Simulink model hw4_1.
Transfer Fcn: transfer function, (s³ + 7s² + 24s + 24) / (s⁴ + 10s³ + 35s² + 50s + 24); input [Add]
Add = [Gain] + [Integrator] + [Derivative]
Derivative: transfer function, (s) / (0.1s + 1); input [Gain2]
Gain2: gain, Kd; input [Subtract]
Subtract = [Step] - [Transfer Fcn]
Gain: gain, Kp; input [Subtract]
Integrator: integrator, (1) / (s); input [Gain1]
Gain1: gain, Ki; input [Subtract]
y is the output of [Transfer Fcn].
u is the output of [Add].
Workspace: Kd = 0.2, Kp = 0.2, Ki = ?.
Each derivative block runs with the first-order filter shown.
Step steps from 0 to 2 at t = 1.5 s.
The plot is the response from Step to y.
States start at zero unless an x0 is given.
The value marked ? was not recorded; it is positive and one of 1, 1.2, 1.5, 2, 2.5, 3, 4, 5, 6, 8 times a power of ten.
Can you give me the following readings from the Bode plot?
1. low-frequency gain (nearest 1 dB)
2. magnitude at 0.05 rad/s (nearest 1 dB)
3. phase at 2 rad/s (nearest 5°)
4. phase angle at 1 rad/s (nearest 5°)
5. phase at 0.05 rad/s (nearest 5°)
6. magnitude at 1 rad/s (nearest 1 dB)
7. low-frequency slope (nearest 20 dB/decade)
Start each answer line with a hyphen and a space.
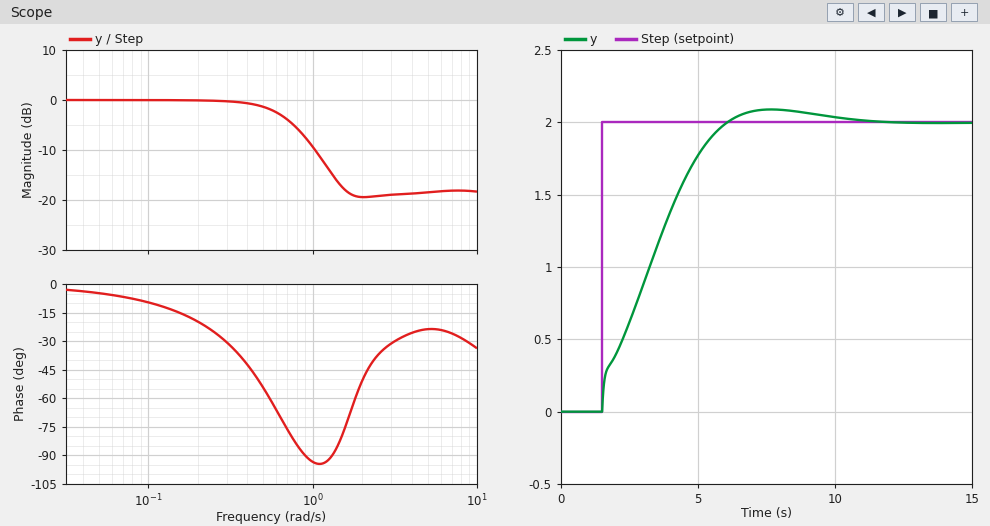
- 0 dB
- 0 dB
- -50°
- -95°
- -5°
- -9 dB
- 0 dB/decade
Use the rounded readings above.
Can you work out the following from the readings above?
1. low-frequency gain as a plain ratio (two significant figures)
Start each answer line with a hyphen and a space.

- 1.0
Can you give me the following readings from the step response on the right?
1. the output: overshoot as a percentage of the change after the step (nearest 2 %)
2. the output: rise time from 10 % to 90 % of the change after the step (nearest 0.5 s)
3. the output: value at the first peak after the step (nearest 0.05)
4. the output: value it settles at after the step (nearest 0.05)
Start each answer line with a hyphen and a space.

- 4 %
- 3.5 s
- 2.10
- 2.00
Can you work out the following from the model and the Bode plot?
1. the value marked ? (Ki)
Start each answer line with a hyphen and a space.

- 0.6
